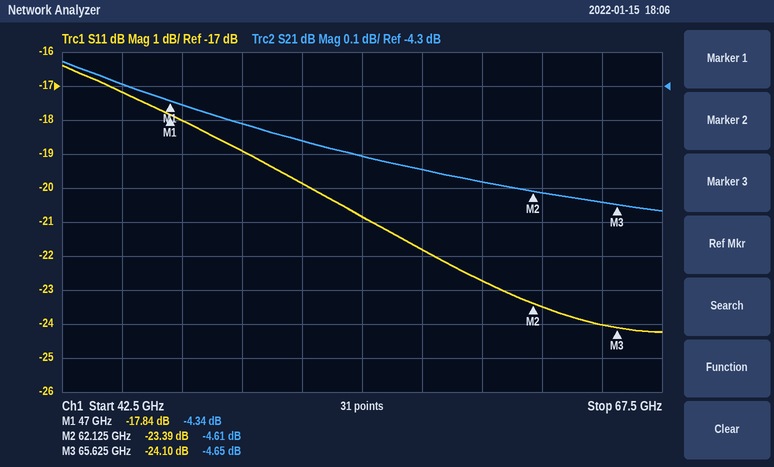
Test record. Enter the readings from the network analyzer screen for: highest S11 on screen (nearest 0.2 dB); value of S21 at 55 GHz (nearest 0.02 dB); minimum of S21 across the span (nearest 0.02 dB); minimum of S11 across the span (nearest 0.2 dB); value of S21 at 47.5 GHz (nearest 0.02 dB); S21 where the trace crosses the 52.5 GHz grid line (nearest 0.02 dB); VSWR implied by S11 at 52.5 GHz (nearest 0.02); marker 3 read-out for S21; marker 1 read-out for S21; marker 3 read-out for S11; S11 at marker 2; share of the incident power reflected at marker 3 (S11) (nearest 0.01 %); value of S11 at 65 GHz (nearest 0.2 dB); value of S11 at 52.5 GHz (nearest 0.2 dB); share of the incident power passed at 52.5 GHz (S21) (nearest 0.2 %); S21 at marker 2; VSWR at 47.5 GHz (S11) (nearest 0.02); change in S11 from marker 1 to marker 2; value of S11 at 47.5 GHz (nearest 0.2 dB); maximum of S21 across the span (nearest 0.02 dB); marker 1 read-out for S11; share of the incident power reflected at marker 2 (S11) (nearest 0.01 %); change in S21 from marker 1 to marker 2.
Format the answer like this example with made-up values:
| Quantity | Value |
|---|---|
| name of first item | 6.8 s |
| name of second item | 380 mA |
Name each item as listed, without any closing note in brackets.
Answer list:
| Quantity | Value |
|---|---|
| highest S11 on screen | -16.4 dB |
| value of S21 at 55 GHz | -4.50 dB |
| minimum of S21 across the span | -4.66 dB |
| minimum of S11 across the span | -24.2 dB |
| value of S21 at 47.5 GHz | -4.36 dB |
| S21 where the trace crosses the 52.5 GHz grid line | -4.46 dB |
| VSWR implied by S11 at 52.5 GHz | 1.22 |
| marker 3 read-out for S21 | -4.65 dB |
| marker 1 read-out for S21 | -4.34 dB |
| marker 3 read-out for S11 | -24.10 dB |
| S11 at marker 2 | -23.39 dB |
| share of the incident power reflected at marker 3 (S11) | 0.39 % |
| value of S11 at 65 GHz | -24.0 dB |
| value of S11 at 52.5 GHz | -19.8 dB |
| share of the incident power passed at 52.5 GHz (S21) | 35.8 % |
| S21 at marker 2 | -4.61 dB |
| VSWR at 47.5 GHz (S11) | 1.28 |
| change in S11 from marker 1 to marker 2 | -5.55 dB |
| value of S11 at 47.5 GHz | -18.0 dB |
| maximum of S21 across the span | -4.22 dB |
| marker 1 read-out for S11 | -17.84 dB |
| share of the incident power reflected at marker 2 (S11) | 0.46 % |
| change in S21 from marker 1 to marker 2 | -0.27 dB |
